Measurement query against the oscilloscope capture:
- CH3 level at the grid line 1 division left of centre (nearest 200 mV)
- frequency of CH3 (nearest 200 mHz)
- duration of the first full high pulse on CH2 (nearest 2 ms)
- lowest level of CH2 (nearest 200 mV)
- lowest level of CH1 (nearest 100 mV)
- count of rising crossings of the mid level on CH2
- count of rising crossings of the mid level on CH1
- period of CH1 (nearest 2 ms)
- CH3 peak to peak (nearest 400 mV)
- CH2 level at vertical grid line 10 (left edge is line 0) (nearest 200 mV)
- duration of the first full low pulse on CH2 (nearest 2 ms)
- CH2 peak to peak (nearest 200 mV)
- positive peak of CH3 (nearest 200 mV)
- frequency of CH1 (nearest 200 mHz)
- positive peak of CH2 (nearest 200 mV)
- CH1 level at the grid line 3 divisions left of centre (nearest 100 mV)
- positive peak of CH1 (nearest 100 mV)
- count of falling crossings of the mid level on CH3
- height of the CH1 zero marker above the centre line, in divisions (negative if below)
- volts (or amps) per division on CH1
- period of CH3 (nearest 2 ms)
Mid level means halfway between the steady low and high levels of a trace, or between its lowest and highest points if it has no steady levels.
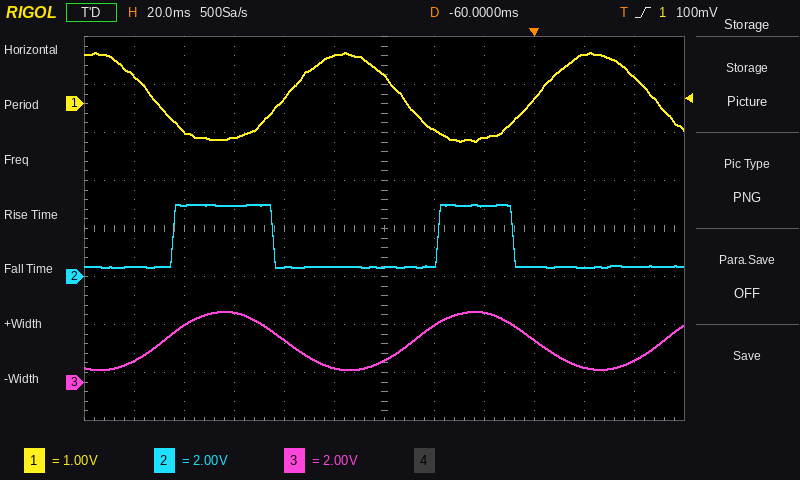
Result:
600 mV
10.0 Hz
40 ms
400 mV
-800 mV
2
2
100 ms
2.4 V
400 mV
66 ms
2.6 V
3.0 V
10.0 Hz
3.0 V
-700 mV
1.1 V
2
+2.6 div
1 V
100 ms
